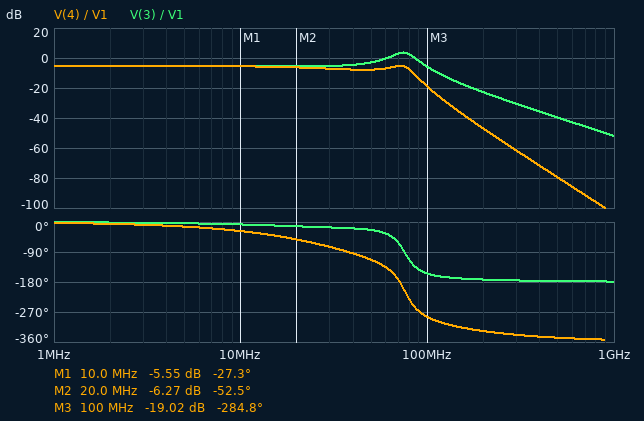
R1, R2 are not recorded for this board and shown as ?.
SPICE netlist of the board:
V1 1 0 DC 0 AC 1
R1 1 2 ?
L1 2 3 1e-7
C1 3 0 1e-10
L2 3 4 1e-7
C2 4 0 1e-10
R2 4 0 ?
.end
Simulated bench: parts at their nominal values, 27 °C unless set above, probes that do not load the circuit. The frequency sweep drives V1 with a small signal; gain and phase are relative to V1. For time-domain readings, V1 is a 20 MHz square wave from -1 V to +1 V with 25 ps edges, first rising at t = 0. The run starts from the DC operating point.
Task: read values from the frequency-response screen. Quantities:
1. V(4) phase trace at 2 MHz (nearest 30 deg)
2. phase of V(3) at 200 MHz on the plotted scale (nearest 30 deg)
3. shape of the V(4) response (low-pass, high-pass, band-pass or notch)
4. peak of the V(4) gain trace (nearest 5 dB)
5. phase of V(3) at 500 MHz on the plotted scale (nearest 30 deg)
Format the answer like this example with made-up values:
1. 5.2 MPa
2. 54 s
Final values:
1. 0 deg
2. -180 deg
3. low-pass
4. -5 dB
5. -180 deg
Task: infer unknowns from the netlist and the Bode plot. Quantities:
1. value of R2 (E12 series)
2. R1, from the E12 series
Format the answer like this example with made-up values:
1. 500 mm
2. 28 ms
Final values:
1. 18 Ω
2. 15 Ω
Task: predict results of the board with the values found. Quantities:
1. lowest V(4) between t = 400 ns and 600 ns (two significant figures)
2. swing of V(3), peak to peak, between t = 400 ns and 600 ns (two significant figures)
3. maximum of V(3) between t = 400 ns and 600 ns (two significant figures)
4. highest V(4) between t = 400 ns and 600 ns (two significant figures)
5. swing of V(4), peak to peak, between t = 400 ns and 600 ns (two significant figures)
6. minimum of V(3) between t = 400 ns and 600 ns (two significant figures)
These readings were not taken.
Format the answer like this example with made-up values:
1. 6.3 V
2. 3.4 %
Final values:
1. -590 mV
2. 1.8 V
3. 900 mV
4. 590 mV
5. 1.2 V
6. -900 mV
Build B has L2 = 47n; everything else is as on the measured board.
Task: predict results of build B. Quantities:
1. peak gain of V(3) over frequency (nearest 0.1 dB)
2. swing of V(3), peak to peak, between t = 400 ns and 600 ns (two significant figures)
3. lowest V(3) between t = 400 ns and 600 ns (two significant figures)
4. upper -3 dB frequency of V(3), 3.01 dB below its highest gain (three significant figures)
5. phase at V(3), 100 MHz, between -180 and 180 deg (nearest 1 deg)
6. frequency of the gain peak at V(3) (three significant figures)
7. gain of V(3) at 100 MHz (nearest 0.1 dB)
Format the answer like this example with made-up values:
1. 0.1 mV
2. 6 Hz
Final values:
1. -2.4 dB
2. 1.3 V
3. -650 mV
4. 115 MHz
5. -92 deg
6. 101 MHz
7. -2.5 dB
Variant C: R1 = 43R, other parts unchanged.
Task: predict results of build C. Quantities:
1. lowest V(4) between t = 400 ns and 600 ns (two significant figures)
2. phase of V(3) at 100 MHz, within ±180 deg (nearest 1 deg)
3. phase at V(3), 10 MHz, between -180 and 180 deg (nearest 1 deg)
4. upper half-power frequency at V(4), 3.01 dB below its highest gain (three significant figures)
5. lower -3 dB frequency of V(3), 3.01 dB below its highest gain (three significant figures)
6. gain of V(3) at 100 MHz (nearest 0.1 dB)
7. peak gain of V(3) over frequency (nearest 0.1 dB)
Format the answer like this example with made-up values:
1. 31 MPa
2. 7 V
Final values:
1. -380 mV
2. -129 deg
3. -1 deg
4. 78.7 MHz
5. 52.0 MHz
6. -8.6 dB
7. -2.0 dB
